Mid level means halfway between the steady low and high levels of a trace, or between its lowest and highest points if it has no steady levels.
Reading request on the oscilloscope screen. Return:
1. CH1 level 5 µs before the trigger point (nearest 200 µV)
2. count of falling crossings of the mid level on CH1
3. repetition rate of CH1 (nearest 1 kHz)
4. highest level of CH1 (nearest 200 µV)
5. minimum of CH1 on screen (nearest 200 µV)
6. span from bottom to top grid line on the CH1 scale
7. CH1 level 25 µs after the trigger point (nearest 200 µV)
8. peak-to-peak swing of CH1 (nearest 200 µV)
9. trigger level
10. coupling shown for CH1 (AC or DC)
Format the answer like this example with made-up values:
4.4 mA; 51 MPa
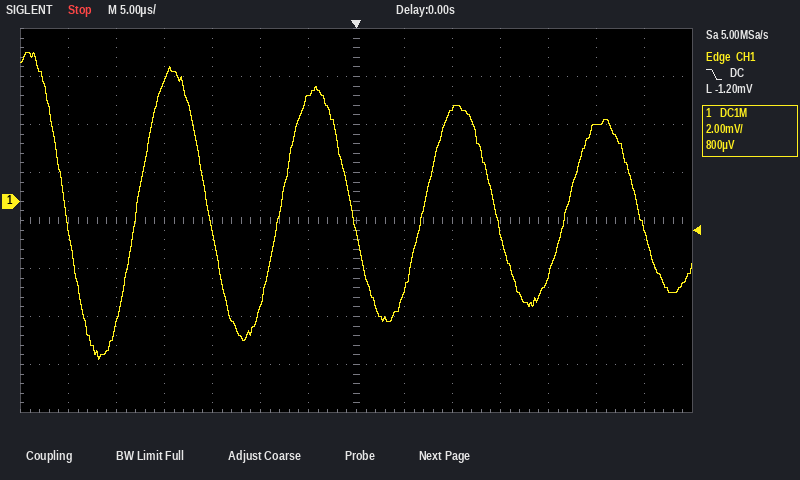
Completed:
4.4 mV; 5; 67 kHz; 6.2 mV; -6.6 mV; 16 mV; 3.2 mV; 12.8 mV; -1.20 mV; DC
